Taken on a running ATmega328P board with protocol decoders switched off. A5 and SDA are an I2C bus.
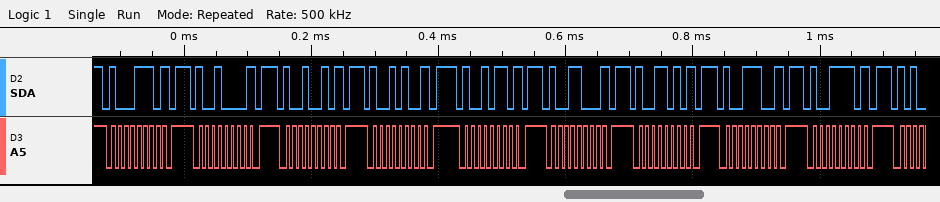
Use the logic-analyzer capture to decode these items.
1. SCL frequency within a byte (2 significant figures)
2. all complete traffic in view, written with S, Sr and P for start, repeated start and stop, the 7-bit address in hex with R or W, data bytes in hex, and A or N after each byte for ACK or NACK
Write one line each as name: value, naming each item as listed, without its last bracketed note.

SCL frequency within a byte: 100 kHz
all complete traffic in view, written with S, Sr and P for start, repeated start and stop, the 7-bit address in hex with R or W, data bytes in hex, and A or N after each byte for ACK or NACK: S 47W N P S 48W N P S 49W N P S 4AW N P S 4BW N P S 4CW N P S 4DW N P S 4EW N P S 4FW N P
